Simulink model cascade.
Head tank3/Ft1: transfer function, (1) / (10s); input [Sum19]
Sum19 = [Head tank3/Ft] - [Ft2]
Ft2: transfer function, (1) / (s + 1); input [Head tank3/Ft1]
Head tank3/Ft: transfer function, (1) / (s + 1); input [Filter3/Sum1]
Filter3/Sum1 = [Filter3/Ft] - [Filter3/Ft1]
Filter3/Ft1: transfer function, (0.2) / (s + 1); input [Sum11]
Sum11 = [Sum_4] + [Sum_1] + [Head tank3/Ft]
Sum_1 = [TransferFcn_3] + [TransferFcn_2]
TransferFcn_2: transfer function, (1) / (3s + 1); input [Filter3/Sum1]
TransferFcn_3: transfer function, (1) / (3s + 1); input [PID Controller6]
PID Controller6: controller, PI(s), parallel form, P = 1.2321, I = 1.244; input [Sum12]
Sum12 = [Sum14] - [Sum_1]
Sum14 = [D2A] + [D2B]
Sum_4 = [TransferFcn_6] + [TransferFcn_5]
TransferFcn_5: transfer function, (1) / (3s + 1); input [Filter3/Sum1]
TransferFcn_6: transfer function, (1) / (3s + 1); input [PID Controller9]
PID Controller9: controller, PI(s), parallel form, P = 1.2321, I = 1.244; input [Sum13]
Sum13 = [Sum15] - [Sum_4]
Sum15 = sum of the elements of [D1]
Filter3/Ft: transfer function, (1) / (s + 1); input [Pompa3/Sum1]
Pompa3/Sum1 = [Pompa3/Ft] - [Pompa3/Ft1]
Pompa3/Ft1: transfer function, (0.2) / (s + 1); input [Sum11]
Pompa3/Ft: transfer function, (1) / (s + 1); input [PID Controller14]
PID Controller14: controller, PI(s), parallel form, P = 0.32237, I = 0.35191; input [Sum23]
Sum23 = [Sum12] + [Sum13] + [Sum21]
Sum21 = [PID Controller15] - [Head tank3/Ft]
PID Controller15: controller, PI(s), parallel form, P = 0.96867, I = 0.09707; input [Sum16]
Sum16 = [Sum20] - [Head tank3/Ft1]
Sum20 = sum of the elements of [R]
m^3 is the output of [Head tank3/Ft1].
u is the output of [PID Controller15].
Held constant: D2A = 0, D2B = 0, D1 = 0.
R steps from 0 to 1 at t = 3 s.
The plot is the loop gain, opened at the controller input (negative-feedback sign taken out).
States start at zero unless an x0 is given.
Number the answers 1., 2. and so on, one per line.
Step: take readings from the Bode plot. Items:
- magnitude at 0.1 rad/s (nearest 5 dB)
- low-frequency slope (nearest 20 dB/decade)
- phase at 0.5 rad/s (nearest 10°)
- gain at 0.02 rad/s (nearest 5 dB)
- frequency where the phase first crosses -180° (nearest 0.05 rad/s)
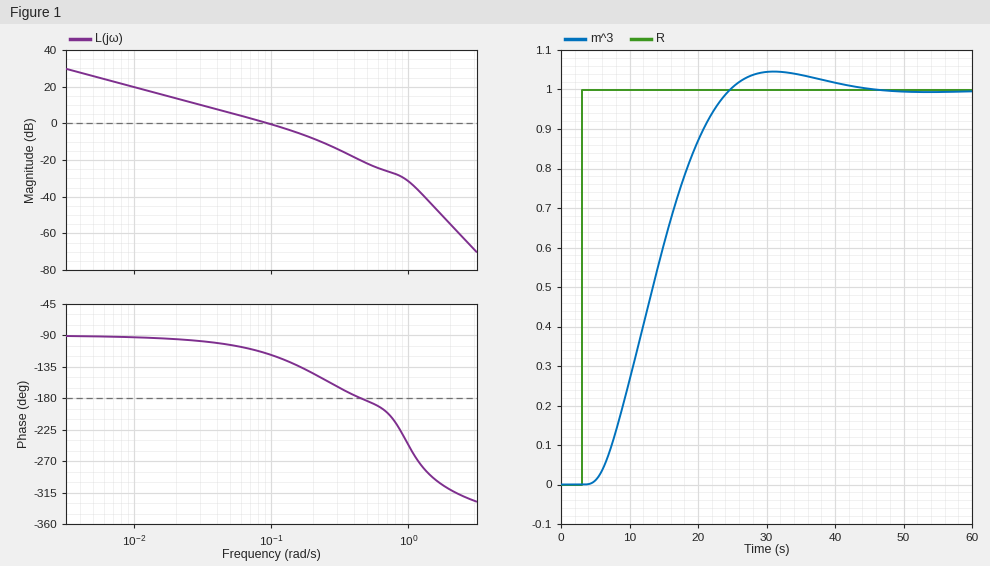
1. 0 dB
2. -20 dB/decade
3. -180°
4. 15 dB
5. 0.45 rad/s
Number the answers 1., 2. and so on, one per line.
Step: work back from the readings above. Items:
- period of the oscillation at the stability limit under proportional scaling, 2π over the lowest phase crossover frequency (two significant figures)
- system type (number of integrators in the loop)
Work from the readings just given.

1. 14 s
2. 1
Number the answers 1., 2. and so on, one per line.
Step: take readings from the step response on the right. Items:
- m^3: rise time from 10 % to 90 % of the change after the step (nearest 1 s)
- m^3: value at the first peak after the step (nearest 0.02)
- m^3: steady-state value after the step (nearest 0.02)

1. 13 s
2. 1.04
3. 1.00
